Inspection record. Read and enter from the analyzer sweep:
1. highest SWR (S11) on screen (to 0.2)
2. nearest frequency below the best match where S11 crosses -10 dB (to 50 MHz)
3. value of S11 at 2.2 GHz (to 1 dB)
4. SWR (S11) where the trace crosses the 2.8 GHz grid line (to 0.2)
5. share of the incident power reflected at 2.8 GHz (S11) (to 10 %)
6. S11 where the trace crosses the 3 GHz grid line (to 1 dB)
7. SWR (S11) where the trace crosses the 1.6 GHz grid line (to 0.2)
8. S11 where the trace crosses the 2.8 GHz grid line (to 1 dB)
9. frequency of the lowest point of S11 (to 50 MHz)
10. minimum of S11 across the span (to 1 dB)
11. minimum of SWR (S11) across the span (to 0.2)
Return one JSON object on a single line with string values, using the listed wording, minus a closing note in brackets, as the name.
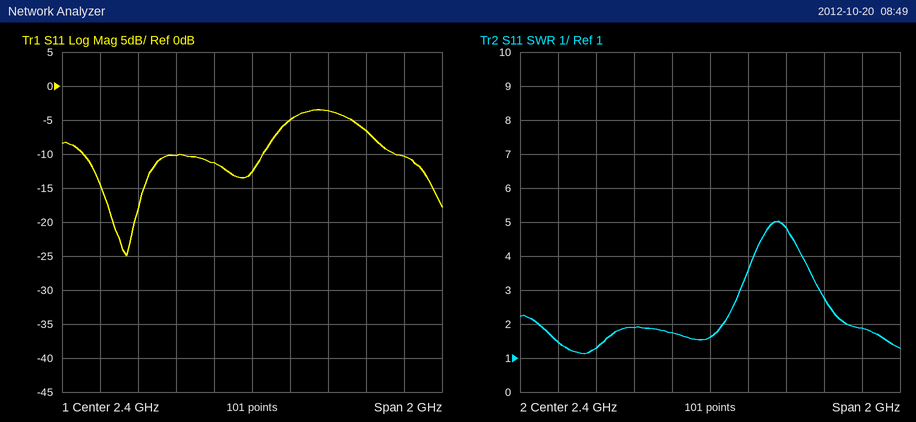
{"highest SWR (S11) on screen": "5.0", "nearest frequency below the best match where S11 crosses -10 dB": "1.50 GHz", "value of S11 at 2.2 GHz": "-11 dB", "SWR (S11) where the trace crosses the 2.8 GHz grid line": "4.8", "share of the incident power reflected at 2.8 GHz (S11)": "40 %", "S11 where the trace crosses the 3 GHz grid line": "-7 dB", "SWR (S11) where the trace crosses the 1.6 GHz grid line": "1.4", "S11 where the trace crosses the 2.8 GHz grid line": "-4 dB", "frequency of the lowest point of S11": "1.75 GHz", "minimum of S11 across the span": "-25 dB", "minimum of SWR (S11) across the span": "1.2"}
